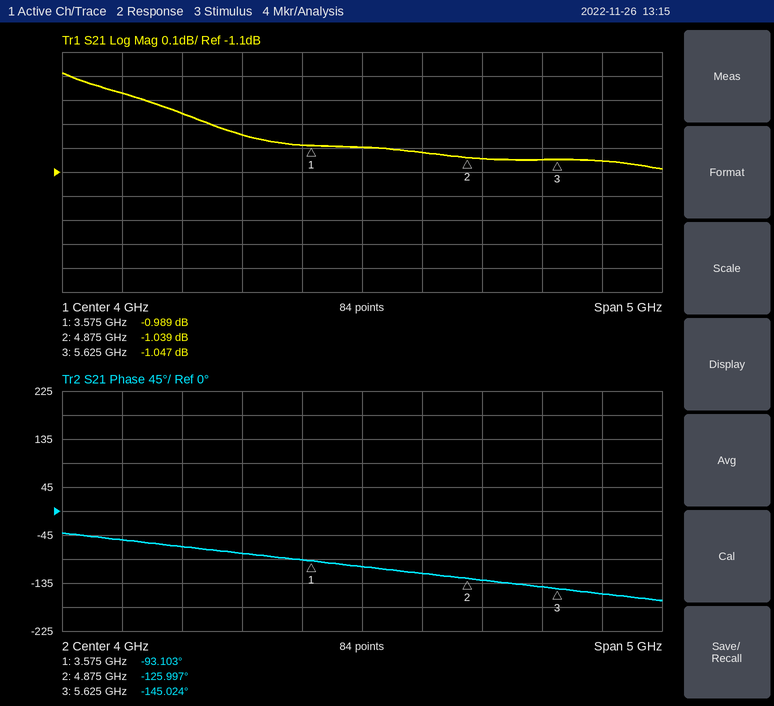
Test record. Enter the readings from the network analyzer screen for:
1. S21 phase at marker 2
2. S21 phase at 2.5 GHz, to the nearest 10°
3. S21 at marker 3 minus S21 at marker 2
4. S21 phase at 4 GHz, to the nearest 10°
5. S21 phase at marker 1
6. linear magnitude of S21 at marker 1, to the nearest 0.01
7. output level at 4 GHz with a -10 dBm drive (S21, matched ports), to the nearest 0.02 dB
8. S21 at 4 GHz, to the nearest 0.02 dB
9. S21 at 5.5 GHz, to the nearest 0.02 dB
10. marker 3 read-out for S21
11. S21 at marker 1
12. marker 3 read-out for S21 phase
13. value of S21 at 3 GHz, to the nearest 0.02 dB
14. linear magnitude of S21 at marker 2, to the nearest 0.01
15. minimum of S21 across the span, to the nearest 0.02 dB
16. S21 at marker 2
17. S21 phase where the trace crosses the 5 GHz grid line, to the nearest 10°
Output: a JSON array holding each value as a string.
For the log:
["-125.997°", "-70°", "-0.008 dB", "-100°", "-93.103°", "0.89", "-11.00 dBm", "-1.00 dB", "-1.04 dB", "-1.047 dB", "-0.989 dB", "-145.024°", "-0.94 dB", "0.89", "-1.08 dB", "-1.039 dB", "-130°"]
